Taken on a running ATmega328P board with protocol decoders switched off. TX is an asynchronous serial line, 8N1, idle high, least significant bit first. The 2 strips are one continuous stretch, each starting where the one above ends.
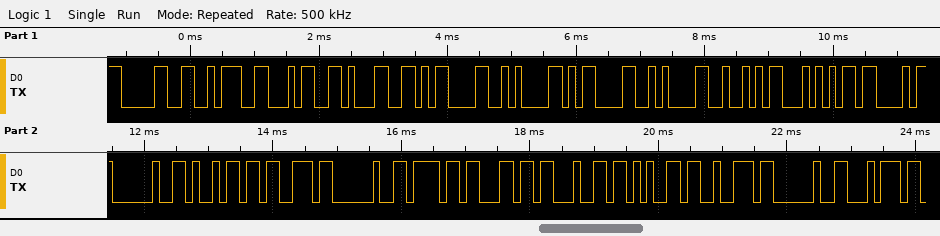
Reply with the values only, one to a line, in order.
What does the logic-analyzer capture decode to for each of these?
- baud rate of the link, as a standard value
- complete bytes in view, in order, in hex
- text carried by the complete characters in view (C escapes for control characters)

9600 baud
0x30 0x3A 0x34 0x31 0x0D 0x0A 0x0D 0x0A 0x52 0x54 0x43 0x20 0x69 0x73 0x20 0x6F 0x6C 0x64 0x65 0x72 0x20 0x74
"0:41\r\n\r\nRTC is older t"
